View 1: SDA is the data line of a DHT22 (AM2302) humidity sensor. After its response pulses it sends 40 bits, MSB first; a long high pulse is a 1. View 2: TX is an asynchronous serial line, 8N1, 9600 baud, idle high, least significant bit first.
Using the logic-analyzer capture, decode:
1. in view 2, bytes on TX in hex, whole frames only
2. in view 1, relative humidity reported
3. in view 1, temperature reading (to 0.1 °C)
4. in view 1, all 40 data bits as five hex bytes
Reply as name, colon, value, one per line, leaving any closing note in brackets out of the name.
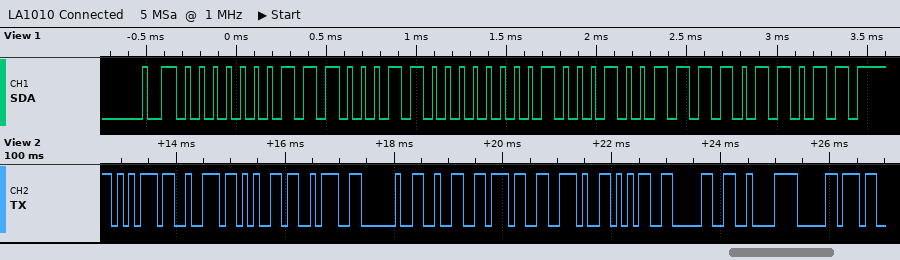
in view 2, bytes on TX in hex, whole frames only: 75 72 65 3A 20 32 37 2E 35 30 C2 B0
in view 1, relative humidity reported: 45.4 %
in view 1, temperature reading: 27.5 °C
in view 1, all 40 data bits as five hex bytes: 01 C6 01 13 DB
